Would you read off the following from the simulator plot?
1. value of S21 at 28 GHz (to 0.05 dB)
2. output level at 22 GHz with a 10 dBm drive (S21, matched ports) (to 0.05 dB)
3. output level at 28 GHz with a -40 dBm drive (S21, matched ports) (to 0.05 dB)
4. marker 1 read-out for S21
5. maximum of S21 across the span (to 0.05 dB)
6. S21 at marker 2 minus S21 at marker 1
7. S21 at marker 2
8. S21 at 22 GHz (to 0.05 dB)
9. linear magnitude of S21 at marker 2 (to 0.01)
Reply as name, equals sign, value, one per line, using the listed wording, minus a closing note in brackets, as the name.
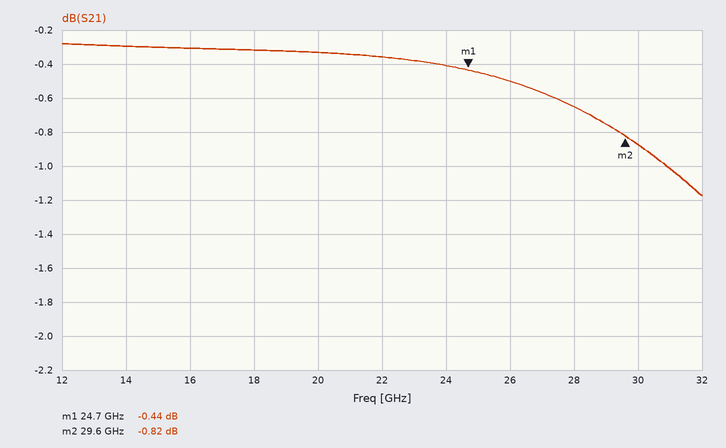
value of S21 at 28 GHz = -0.65 dB
output level at 22 GHz with a 10 dBm drive (S21, matched ports) = 9.65 dBm
output level at 28 GHz with a -40 dBm drive (S21, matched ports) = -40.65 dBm
marker 1 read-out for S21 = -0.44 dB
maximum of S21 across the span = -0.30 dB
S21 at marker 2 minus S21 at marker 1 = -0.38 dB
S21 at marker 2 = -0.82 dB
S21 at 22 GHz = -0.35 dB
linear magnitude of S21 at marker 2 = 0.91
